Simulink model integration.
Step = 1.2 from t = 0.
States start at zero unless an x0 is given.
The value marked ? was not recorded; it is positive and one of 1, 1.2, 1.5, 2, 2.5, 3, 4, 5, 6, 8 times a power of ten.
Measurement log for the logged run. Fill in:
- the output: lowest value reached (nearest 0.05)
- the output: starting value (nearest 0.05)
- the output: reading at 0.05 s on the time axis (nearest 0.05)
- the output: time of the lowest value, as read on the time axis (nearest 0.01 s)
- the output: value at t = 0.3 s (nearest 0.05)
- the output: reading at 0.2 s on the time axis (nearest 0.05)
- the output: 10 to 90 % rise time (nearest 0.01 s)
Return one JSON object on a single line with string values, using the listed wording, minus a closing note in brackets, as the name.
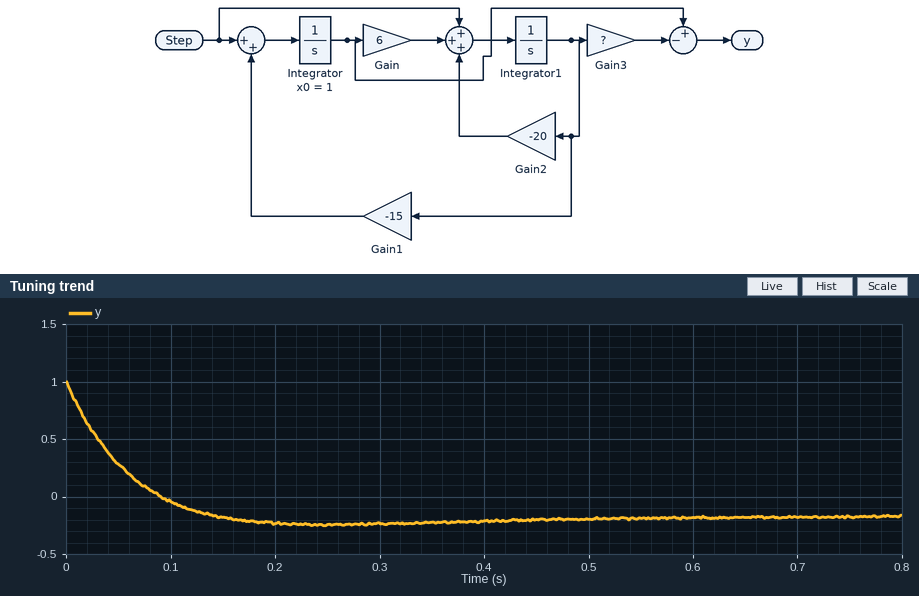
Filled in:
{"the output: lowest value reached": "-0.25", "the output: starting value": "1.00", "the output: reading at 0.05 s on the time axis": "0.30", "the output: time of the lowest value, as read on the time axis": "0.25 s", "the output: value at t = 0.3 s": "-0.25", "the output: reading at 0.2 s on the time axis": "-0.25", "the output: 10 to 90 % rise time": "0.10 s"}
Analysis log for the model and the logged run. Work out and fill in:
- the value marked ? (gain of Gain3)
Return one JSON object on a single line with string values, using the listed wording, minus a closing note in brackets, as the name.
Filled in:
{"the value marked ?": "3"}
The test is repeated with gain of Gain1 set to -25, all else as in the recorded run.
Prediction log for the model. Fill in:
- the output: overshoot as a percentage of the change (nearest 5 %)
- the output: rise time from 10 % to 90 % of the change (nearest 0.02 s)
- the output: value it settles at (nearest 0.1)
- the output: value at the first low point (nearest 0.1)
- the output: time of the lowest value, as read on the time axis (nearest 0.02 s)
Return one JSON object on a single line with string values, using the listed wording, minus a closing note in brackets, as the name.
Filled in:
{"the output: overshoot as a percentage of the change": "10 %", "the output: rise time from 10 % to 90 % of the change": "0.08 s", "the output: value it settles at": "-0.2", "the output: value at the first low point": "-0.3", "the output: time of the lowest value, as read on the time axis": "0.20 s"}
